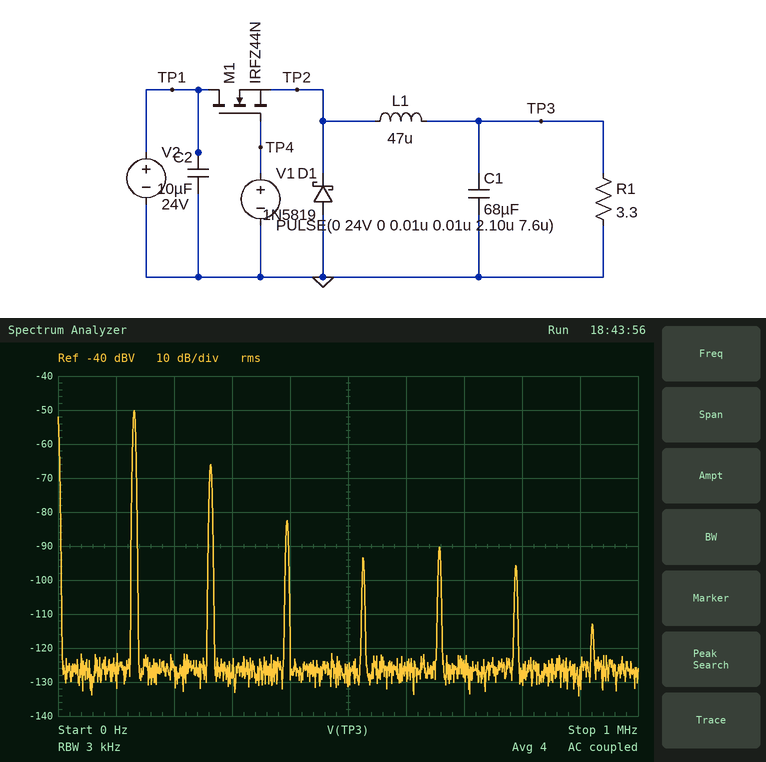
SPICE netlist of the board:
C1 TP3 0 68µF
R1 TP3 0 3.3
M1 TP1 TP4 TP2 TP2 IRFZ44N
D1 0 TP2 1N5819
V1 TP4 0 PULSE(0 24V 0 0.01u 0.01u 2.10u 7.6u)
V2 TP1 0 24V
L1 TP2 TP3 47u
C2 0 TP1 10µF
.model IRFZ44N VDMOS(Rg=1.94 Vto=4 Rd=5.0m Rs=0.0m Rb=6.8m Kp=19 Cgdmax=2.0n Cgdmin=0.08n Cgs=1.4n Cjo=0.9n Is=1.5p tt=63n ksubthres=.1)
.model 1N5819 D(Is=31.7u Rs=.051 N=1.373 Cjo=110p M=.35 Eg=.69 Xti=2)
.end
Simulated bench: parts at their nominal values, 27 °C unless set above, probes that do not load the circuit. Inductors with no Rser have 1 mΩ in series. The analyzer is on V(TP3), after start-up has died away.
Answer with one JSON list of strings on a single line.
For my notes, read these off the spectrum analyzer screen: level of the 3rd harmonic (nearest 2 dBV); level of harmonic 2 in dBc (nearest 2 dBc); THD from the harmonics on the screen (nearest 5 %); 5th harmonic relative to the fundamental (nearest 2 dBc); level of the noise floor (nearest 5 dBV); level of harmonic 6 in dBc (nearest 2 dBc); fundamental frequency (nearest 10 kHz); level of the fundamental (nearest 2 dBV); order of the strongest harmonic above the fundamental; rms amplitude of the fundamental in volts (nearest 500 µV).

["-82 dBV", "-16 dBc", "15 %", "-40 dBc", "-125 dBV", "-46 dBc", "130 kHz", "-50 dBV", "2", "3.0 mV"]
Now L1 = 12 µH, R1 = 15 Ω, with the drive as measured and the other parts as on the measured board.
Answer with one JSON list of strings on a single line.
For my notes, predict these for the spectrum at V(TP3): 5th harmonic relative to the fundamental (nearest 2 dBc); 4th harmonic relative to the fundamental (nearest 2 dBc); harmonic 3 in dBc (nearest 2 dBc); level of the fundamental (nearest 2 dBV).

["-38 dBc", "-42 dBc", "-36 dBc", "-40 dBV"]
